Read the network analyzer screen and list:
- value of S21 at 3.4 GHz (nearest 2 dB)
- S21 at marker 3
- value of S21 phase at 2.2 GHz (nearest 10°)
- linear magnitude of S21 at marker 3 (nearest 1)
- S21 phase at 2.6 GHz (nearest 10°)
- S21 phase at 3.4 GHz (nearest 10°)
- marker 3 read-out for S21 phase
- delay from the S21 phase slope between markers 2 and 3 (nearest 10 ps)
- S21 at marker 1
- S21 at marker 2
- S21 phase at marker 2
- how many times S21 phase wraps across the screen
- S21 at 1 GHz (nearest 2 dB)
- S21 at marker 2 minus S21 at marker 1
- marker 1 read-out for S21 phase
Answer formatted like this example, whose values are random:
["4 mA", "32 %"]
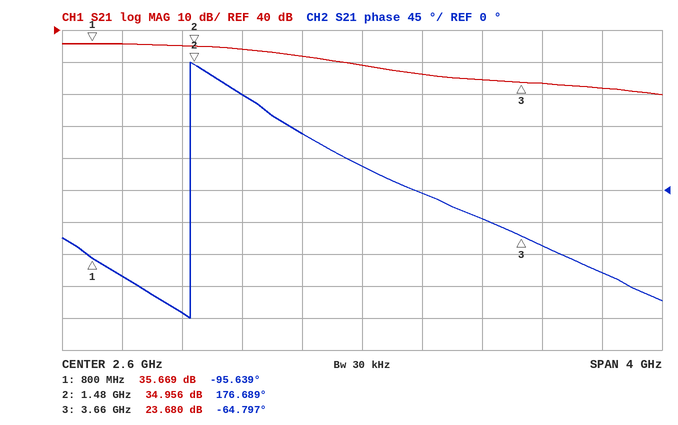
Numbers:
["24 dB", "23.680 dB", "80°", "15", "30°", "-40°", "-64.797°", "310 ps", "35.669 dB", "34.956 dB", "176.689°", "1", "36 dB", "-0.713 dB", "-95.639°"]
